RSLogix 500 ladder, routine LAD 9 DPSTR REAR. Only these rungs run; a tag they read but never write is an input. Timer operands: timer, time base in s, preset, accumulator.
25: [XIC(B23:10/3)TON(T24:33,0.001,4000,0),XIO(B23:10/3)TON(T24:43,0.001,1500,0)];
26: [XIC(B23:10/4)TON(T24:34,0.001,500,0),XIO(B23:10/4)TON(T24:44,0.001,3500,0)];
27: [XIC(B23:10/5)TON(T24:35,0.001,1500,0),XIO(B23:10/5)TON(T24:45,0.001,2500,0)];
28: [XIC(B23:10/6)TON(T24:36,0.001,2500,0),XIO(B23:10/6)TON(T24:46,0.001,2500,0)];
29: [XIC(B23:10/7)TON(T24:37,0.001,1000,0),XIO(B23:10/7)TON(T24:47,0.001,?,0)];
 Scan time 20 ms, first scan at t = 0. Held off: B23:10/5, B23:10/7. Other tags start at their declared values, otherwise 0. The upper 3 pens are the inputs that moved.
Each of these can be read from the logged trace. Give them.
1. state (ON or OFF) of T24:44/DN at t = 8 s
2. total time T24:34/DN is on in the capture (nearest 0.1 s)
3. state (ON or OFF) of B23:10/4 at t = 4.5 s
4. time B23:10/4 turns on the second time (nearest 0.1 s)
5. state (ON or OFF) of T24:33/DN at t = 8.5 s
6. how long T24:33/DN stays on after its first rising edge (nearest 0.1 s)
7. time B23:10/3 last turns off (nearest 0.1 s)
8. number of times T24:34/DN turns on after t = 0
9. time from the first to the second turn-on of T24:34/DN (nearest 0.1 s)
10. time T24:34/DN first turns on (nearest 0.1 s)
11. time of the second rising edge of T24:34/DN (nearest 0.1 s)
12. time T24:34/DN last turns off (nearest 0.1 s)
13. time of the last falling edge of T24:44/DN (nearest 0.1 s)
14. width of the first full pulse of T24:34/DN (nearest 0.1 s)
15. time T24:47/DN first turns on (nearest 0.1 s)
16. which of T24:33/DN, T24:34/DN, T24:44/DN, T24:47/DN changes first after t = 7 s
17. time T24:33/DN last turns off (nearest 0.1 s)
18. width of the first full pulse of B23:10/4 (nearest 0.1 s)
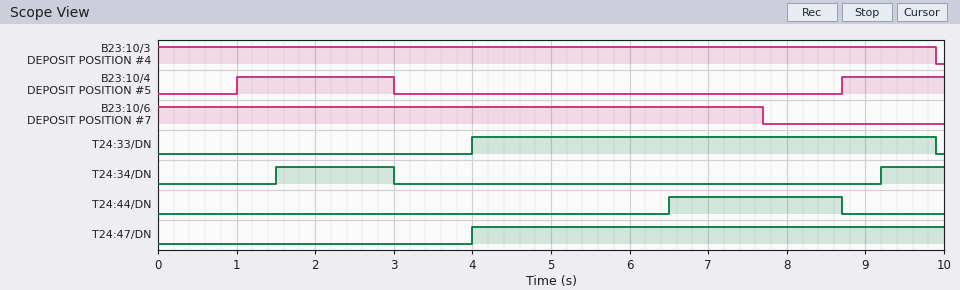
ON
2.3 s
OFF
8.7 s
ON
5.9 s
9.9 s
2
7.7 s
1.5 s
9.2 s
3.0 s
8.7 s
1.5 s
4.0 s
T24:44/DN
9.9 s
2.0 s
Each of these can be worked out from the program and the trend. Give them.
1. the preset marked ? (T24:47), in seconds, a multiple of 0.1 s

4.0 s
